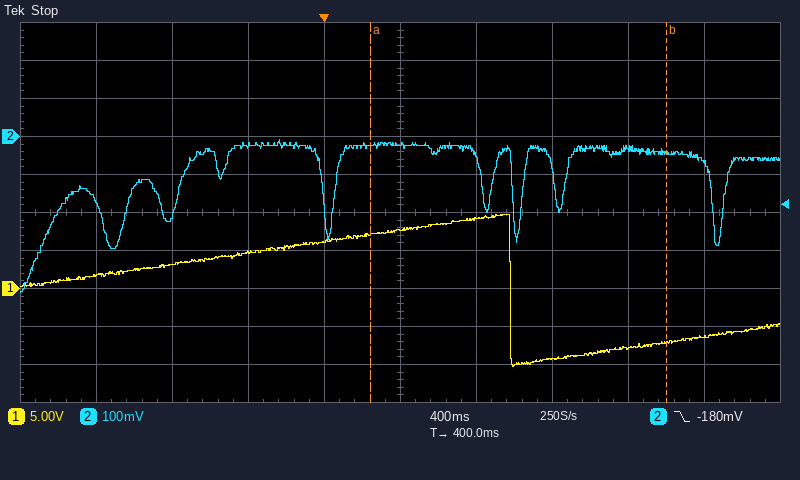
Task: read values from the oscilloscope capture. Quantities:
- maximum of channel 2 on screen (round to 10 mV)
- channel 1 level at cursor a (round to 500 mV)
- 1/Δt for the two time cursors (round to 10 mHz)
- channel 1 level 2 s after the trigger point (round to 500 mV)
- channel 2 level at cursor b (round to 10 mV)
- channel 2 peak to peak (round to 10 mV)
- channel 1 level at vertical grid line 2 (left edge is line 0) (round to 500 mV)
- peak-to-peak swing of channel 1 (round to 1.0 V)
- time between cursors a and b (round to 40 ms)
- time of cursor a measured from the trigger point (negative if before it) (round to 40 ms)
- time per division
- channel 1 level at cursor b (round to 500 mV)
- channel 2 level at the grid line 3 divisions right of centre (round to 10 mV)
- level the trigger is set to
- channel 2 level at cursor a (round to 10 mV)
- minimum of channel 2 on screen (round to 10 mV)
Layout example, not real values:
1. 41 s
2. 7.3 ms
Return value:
1. -10 mV
2. 7.0 V
3. 640 mHz
4. -6.5 V
5. -40 mV
6. 400 mV
7. 3.0 V
8. 20.0 V
9. 1.56 s
10. +240 ms
11. 400 ms
12. -7.0 V
13. -30 mV
14. -180 mV
15. -20 mV
16. -410 mV
